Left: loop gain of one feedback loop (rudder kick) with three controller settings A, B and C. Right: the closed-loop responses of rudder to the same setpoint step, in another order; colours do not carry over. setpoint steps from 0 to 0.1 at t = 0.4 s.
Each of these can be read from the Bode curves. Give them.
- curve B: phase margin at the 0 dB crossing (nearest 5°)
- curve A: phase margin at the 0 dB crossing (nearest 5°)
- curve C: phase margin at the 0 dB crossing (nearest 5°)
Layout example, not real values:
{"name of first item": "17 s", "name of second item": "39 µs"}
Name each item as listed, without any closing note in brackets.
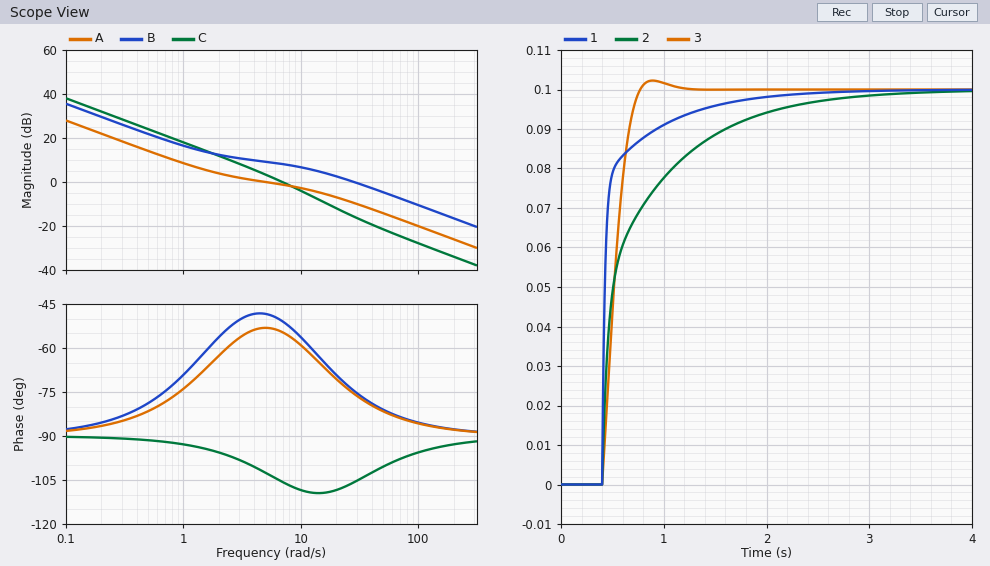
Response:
{"curve B: phase margin at the 0 dB crossing": "105°", "curve A: phase margin at the 0 dB crossing": "125°", "curve C: phase margin at the 0 dB crossing": "75°"}
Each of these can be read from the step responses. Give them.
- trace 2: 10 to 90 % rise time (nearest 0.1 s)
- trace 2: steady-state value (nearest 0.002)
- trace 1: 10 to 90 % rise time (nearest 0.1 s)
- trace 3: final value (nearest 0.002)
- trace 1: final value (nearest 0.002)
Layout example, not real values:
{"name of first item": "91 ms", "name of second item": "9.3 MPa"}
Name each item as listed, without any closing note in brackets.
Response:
{"trace 2: 10 to 90 % rise time": "1.2 s", "trace 2: steady-state value": "0.100", "trace 1: 10 to 90 % rise time": "0.5 s", "trace 3: final value": "0.100", "trace 1: final value": "0.100"}
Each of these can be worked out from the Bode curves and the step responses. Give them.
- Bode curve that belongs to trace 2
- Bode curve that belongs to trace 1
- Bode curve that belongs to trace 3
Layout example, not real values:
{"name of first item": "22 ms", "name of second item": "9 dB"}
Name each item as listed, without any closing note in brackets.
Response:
{"Bode curve that belongs to trace 2": "A", "Bode curve that belongs to trace 1": "B", "Bode curve that belongs to trace 3": "C"}
